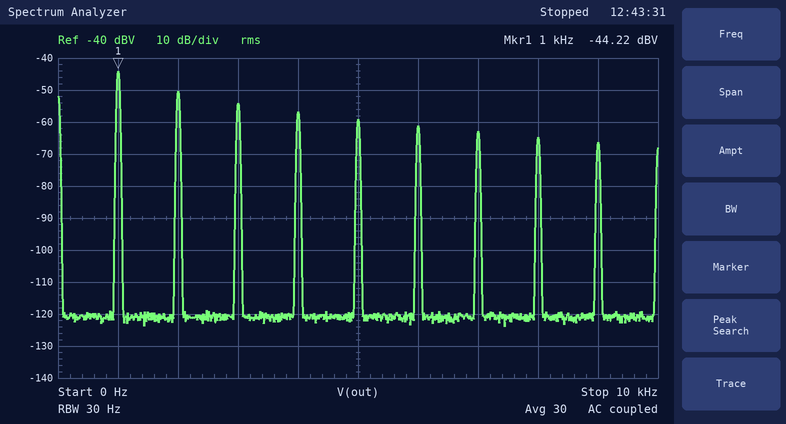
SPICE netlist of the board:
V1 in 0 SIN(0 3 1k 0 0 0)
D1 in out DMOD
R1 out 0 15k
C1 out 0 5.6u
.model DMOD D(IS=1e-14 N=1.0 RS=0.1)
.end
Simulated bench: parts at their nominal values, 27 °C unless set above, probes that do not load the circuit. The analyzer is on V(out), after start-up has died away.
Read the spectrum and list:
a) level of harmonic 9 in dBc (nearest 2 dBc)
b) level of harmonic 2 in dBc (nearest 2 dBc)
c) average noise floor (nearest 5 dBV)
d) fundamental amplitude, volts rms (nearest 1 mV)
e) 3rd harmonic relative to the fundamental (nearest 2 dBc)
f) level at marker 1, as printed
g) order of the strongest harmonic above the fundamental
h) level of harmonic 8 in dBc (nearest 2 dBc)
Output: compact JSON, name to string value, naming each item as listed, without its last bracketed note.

{"level of harmonic 9 in dBc": "-22 dBc", "level of harmonic 2 in dBc": "-6 dBc", "average noise floor": "-120 dBV", "fundamental amplitude, volts rms": "6 mV", "3rd harmonic relative to the fundamental": "-10 dBc", "level at marker 1, as printed": "-44.22 dBV", "order of the strongest harmonic above the fundamental": "2", "level of harmonic 8 in dBc": "-20 dBc"}
